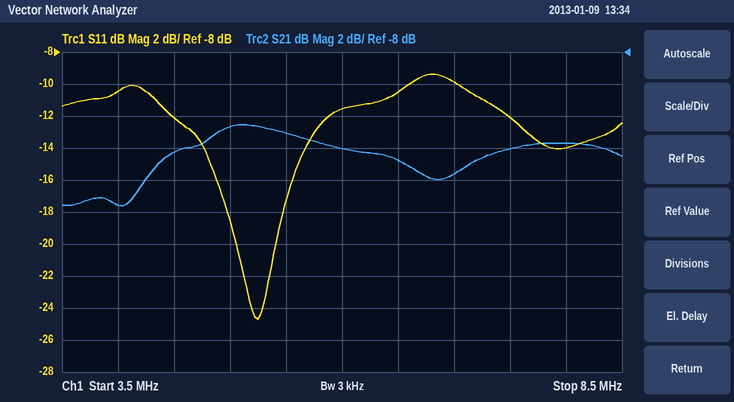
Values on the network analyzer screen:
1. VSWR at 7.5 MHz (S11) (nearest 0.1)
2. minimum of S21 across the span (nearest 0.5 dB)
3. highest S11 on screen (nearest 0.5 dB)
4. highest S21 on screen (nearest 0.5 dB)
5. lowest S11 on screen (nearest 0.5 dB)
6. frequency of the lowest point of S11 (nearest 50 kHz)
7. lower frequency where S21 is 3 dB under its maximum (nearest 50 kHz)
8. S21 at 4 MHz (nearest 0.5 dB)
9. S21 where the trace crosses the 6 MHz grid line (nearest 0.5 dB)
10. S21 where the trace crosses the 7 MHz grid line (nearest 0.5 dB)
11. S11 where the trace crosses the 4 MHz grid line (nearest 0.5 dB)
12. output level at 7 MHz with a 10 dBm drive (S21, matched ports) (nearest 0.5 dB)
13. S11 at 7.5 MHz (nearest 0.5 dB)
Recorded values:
1.7
-17.5 dB
-9.5 dB
-12.5 dB
-24.5 dB
5.25 MHz
4.30 MHz
-17.5 dB
-14.0 dB
-15.5 dB
-10.5 dB
-5.5 dBm
-12.0 dB
